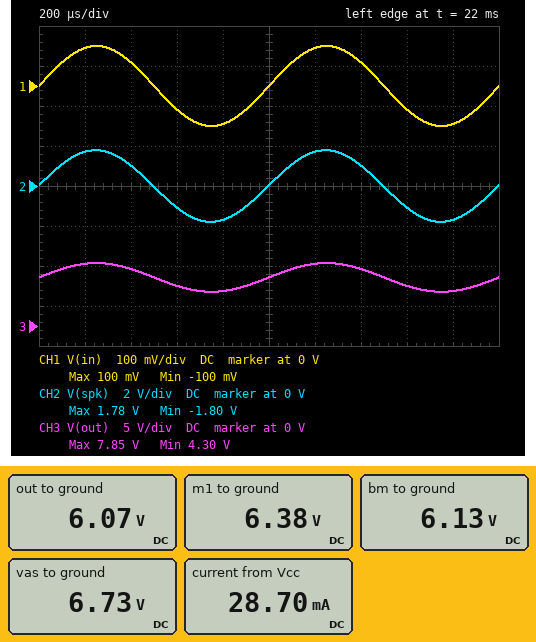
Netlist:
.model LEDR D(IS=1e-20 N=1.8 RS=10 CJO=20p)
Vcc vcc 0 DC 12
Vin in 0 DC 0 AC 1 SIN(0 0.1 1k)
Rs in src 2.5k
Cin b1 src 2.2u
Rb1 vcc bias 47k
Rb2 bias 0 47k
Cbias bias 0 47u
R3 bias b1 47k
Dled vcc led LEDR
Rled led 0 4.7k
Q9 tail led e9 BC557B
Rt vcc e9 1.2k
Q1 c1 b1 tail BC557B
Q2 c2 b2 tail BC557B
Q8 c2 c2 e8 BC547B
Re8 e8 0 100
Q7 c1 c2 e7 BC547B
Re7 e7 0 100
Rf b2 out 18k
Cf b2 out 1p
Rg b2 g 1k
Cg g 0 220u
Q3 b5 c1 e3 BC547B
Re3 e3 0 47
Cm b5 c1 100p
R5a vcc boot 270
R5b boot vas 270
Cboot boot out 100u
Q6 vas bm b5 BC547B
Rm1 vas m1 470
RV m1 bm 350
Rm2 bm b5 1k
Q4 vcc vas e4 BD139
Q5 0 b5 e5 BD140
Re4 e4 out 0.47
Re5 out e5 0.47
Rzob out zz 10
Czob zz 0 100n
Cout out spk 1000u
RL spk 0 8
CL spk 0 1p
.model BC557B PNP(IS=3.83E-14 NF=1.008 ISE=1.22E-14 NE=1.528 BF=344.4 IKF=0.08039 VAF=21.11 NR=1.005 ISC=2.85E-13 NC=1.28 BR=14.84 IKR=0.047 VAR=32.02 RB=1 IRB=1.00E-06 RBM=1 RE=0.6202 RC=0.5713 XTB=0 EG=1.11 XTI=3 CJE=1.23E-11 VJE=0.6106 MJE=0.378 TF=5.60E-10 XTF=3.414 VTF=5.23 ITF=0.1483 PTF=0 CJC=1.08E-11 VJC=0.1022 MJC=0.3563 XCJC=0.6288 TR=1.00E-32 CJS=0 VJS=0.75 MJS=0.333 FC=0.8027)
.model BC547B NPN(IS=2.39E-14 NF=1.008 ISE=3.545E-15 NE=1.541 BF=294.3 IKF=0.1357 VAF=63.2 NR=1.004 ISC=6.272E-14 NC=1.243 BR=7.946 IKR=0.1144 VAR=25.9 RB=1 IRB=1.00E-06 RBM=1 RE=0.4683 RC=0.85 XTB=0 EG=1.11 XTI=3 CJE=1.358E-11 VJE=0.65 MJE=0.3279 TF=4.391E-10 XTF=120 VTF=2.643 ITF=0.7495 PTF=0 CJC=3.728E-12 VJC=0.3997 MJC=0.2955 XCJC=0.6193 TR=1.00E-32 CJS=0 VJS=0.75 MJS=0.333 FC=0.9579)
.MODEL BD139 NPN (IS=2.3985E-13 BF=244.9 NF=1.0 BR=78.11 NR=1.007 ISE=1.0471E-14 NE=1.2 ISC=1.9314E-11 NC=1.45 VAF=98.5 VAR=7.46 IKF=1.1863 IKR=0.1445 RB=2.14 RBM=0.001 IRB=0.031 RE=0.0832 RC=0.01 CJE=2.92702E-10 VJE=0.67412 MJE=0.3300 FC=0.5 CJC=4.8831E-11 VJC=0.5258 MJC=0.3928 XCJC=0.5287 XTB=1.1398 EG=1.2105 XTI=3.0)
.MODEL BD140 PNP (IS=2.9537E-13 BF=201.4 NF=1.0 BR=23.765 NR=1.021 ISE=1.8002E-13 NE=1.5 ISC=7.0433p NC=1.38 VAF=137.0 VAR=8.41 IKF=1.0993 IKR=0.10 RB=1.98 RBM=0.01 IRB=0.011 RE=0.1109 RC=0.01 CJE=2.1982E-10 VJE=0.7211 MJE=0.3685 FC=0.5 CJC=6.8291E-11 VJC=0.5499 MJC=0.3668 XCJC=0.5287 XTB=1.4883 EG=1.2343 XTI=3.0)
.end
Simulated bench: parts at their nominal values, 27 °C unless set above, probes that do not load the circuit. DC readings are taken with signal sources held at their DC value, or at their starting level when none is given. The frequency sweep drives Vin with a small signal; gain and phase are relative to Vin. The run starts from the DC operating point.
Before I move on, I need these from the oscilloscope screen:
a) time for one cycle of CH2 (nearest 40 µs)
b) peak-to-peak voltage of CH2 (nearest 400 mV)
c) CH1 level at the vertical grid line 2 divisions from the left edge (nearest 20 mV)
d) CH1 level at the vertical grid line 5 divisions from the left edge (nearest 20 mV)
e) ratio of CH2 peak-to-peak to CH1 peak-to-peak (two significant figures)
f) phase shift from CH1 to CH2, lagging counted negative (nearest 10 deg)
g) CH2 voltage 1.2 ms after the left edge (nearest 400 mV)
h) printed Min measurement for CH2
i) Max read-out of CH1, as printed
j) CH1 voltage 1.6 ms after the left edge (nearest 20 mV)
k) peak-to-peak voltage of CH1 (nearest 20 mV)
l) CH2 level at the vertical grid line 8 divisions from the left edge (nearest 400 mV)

1.00 ms
3.6 V
60 mV
0 V
18
0 deg
1.6 V
-1.80 V
100 mV
-60 mV
200 mV
-1.2 V
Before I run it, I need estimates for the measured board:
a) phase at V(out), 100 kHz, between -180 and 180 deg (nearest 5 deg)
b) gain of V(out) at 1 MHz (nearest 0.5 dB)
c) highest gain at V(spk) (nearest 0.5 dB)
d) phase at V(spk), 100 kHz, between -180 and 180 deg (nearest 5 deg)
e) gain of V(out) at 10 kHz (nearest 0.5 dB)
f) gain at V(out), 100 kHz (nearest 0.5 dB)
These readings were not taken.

-5 deg
24.0 dB
25.0 dB
-5 deg
25.0 dB
25.0 dB
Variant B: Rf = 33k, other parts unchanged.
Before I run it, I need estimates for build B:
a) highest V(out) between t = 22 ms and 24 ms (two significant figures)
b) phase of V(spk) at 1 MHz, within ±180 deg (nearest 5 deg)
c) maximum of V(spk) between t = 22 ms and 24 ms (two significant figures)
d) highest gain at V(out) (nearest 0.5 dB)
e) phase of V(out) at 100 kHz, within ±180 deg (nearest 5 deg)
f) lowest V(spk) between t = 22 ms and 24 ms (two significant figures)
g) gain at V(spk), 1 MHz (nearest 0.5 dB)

9.2 V
-95 deg
3.2 V
30.0 dB
-10 deg
-3.2 V
24.5 dB
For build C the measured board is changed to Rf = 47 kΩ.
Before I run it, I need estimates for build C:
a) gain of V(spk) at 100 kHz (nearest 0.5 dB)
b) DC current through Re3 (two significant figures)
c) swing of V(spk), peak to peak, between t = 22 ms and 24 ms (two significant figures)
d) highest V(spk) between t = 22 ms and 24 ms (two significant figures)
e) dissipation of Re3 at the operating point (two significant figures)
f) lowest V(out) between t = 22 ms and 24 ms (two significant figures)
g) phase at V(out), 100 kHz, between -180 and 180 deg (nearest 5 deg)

33.0 dB
9.9 mA
8.6 V
4.4 V
4.6 mW
1.9 V
-15 deg
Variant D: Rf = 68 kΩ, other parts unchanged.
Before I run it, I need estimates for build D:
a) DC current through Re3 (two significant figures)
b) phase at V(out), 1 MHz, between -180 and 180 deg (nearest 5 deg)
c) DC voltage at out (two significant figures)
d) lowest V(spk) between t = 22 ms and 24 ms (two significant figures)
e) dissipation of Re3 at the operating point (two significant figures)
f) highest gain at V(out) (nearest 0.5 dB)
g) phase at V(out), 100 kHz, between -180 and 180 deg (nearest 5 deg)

9.9 mA
-110 deg
6.0 V
-4.5 V
4.6 mW
36.0 dB
-20 deg
